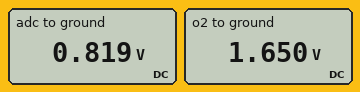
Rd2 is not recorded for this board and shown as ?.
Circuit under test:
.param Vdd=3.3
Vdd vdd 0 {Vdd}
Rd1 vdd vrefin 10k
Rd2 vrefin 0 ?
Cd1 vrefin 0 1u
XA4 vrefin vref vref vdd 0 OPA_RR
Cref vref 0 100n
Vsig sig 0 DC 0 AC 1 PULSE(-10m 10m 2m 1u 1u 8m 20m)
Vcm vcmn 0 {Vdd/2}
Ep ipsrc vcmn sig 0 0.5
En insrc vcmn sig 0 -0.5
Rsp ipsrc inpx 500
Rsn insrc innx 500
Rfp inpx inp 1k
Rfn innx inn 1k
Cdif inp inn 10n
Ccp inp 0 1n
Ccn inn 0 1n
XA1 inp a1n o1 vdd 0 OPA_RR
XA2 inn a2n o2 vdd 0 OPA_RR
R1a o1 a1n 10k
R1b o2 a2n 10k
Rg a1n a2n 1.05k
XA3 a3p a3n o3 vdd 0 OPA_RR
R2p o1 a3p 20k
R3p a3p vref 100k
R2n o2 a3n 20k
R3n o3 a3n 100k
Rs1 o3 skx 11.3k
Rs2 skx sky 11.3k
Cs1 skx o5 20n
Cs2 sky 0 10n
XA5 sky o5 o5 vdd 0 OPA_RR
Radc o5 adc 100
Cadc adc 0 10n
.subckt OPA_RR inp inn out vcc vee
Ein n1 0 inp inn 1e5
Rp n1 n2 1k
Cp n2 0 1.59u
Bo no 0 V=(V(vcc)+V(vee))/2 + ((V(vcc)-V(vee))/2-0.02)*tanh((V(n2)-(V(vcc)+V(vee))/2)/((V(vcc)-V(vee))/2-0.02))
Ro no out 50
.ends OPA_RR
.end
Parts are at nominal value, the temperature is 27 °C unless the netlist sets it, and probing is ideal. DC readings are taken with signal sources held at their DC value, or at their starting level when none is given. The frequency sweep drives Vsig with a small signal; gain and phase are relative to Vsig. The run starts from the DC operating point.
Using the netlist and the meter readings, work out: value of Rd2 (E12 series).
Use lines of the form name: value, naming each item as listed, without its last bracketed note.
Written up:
value of Rd2: 3.3 kΩ
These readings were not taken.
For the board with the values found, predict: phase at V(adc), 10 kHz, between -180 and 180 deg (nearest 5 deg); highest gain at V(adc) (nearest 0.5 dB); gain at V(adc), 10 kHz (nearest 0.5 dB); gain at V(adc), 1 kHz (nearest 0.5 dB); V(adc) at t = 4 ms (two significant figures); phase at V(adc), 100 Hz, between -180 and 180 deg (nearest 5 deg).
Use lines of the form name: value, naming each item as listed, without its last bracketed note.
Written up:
phase at V(adc), 10 kHz, between -180 and 180 deg: 120 deg
highest gain at V(adc): 40.0 dB
gain at V(adc), 10 kHz: -7.0 dB
gain at V(adc), 1 kHz: 37.0 dB
V(adc) at t = 4 ms: 1.8 V
phase at V(adc), 100 Hz, between -180 and 180 deg: -10 deg
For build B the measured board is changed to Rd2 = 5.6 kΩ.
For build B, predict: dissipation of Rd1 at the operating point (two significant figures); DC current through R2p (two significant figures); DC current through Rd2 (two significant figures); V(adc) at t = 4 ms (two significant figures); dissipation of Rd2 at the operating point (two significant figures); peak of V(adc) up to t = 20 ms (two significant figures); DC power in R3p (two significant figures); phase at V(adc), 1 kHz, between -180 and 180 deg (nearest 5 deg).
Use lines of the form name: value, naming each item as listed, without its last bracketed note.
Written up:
dissipation of Rd1 at the operating point: 450 µW
DC current through R2p: 3.9 µA
DC current through Rd2: 210 µA
V(adc) at t = 4 ms: 2.2 V
dissipation of Rd2 at the operating point: 250 µW
peak of V(adc) up to t = 20 ms: 2.3 V
DC power in R3p: 1.5 µW
phase at V(adc), 1 kHz, between -180 and 180 deg: -100 deg
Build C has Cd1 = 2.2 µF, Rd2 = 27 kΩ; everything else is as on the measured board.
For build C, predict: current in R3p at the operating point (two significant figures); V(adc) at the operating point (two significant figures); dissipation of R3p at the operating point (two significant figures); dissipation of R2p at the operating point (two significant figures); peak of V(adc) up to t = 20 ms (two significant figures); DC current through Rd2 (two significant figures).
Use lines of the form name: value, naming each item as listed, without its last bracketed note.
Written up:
current in R3p at the operating point: 6.3 µA
V(adc) at the operating point: 2.4 V
dissipation of R3p at the operating point: 4.0 µW
dissipation of R2p at the operating point: 800 nW
peak of V(adc) up to t = 20 ms: 3.3 V
DC current through Rd2: 89 µA
